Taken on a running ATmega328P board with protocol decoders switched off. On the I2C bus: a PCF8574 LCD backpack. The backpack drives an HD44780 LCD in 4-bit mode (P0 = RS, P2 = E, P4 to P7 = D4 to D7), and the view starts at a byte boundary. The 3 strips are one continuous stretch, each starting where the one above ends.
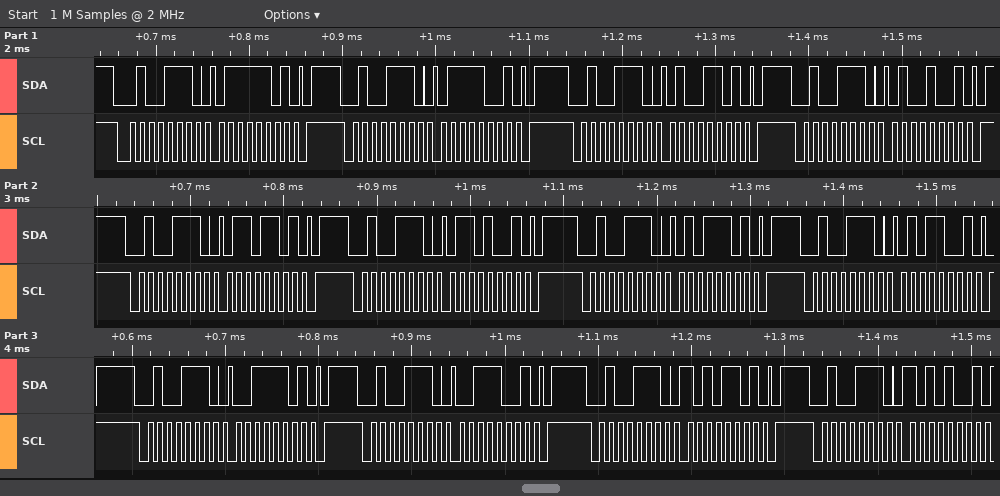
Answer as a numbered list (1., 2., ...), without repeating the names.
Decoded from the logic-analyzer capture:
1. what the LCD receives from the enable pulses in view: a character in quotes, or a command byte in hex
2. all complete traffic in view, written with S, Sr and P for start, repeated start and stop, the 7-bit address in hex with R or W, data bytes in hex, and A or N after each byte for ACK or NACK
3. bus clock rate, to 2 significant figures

1. 't' 'e' ':'
2. S 27W A 7D A P S 27W A 79 A P S 27W A 4D A P S 27W A 49 A P S 27W A 6D A P S 27W A 69 A P S 27W A 5D A P S 27W A 59 A P S 27W A 3D A P S 27W A 39 A P S 27W A AD A P S 27W A A9 A
3. 100 kHz
